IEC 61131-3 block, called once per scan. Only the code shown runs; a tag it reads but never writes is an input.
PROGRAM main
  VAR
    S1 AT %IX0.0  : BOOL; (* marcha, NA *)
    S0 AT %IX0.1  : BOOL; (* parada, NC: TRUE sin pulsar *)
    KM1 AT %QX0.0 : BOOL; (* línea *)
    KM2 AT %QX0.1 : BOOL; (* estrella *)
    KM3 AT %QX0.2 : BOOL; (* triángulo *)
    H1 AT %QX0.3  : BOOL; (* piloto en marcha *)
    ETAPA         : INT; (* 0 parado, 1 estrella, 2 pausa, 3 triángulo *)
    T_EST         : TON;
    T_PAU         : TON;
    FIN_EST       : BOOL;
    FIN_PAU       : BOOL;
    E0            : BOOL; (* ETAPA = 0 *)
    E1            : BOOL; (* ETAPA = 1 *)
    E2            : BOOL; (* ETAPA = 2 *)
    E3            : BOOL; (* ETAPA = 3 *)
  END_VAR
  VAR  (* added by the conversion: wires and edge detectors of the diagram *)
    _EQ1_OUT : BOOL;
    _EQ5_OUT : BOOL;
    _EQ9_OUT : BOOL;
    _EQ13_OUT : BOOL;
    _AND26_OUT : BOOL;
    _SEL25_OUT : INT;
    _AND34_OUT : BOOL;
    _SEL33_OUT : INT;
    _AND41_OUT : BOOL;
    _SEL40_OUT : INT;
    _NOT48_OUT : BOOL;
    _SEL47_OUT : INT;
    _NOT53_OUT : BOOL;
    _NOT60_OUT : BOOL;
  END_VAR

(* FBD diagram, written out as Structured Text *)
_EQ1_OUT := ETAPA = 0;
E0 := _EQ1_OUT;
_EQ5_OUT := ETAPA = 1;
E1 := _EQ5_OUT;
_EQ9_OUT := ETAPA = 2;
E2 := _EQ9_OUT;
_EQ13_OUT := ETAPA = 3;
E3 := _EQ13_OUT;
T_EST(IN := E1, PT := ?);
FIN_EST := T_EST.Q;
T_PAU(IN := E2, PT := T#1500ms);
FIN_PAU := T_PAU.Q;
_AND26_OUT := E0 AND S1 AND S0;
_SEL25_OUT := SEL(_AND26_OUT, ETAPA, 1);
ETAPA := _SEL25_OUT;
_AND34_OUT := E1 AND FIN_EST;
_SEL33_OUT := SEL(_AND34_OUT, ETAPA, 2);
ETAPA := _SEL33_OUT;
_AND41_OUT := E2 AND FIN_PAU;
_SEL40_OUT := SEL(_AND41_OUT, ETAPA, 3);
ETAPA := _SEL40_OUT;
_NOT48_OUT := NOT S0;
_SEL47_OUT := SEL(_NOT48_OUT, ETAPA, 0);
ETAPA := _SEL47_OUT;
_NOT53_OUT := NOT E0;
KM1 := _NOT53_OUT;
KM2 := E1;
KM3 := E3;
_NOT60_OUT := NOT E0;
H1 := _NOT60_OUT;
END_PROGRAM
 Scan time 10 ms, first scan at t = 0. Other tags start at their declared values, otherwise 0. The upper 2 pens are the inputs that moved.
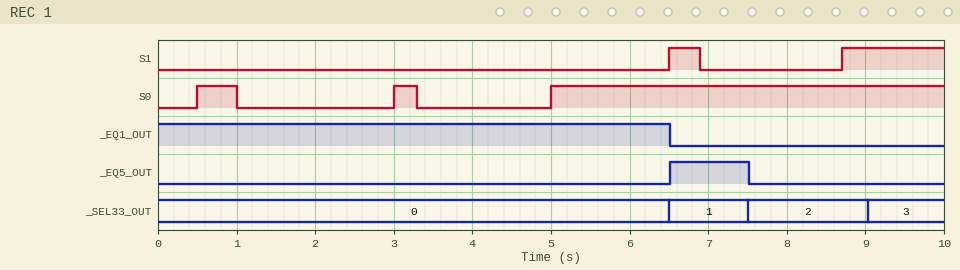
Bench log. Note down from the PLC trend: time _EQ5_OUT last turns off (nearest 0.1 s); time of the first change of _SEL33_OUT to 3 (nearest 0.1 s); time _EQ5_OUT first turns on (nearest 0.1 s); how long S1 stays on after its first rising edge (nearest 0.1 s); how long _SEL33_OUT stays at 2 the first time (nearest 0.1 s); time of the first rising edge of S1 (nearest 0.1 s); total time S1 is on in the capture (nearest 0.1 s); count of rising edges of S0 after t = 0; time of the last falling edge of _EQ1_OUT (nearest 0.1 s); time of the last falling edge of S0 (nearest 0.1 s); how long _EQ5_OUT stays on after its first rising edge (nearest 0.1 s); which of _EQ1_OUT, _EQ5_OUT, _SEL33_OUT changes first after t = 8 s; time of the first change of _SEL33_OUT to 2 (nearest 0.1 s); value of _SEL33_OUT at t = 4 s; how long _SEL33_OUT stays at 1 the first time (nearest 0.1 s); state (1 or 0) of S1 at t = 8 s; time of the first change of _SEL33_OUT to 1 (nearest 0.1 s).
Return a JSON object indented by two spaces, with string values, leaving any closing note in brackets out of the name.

{
  "time _EQ5_OUT last turns off": "7.5 s",
  "time of the first change of _SEL33_OUT to 3": "9.0 s",
  "time _EQ5_OUT first turns on": "6.5 s",
  "how long S1 stays on after its first rising edge": "0.4 s",
  "how long _SEL33_OUT stays at 2 the first time": "1.5 s",
  "time of the first rising edge of S1": "6.5 s",
  "total time S1 is on in the capture": "1.7 s",
  "count of rising edges of S0 after t = 0": "3",
  "time of the last falling edge of _EQ1_OUT": "6.5 s",
  "time of the last falling edge of S0": "3.3 s",
  "how long _EQ5_OUT stays on after its first rising edge": "1.0 s",
  "which of _EQ1_OUT, _EQ5_OUT, _SEL33_OUT changes first after t = 8 s": "_SEL33_OUT",
  "time of the first change of _SEL33_OUT to 2": "7.5 s",
  "value of _SEL33_OUT at t = 4 s": "0",
  "how long _SEL33_OUT stays at 1 the first time": "1.0 s",
  "state (1 or 0) of S1 at t = 8 s": "0",
  "time of the first change of _SEL33_OUT to 1": "6.5 s"
}
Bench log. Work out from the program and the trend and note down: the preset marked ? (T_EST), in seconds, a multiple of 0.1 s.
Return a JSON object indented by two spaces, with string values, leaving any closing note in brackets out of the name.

{
  "the preset marked ? (T_EST), in seconds, a multiple of 0.1 s": "1.0 s"
}
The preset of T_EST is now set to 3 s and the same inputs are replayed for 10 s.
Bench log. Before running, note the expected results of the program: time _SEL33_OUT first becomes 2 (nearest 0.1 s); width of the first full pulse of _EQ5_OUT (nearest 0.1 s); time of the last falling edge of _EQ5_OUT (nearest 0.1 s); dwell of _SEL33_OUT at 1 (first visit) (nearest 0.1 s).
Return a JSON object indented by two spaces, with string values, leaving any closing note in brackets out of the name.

{
  "time _SEL33_OUT first becomes 2": "9.5 s",
  "width of the first full pulse of _EQ5_OUT": "3.0 s",
  "time of the last falling edge of _EQ5_OUT": "9.5 s",
  "dwell of _SEL33_OUT at 1 (first visit)": "3.0 s"
}
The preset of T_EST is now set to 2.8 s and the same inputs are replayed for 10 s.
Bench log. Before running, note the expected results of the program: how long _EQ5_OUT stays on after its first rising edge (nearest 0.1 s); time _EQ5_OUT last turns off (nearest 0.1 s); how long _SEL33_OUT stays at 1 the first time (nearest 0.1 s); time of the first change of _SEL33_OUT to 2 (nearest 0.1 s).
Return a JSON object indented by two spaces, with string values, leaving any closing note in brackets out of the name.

{
  "how long _EQ5_OUT stays on after its first rising edge": "2.8 s",
  "time _EQ5_OUT last turns off": "9.3 s",
  "how long _SEL33_OUT stays at 1 the first time": "2.8 s",
  "time of the first change of _SEL33_OUT to 2": "9.3 s"
}
